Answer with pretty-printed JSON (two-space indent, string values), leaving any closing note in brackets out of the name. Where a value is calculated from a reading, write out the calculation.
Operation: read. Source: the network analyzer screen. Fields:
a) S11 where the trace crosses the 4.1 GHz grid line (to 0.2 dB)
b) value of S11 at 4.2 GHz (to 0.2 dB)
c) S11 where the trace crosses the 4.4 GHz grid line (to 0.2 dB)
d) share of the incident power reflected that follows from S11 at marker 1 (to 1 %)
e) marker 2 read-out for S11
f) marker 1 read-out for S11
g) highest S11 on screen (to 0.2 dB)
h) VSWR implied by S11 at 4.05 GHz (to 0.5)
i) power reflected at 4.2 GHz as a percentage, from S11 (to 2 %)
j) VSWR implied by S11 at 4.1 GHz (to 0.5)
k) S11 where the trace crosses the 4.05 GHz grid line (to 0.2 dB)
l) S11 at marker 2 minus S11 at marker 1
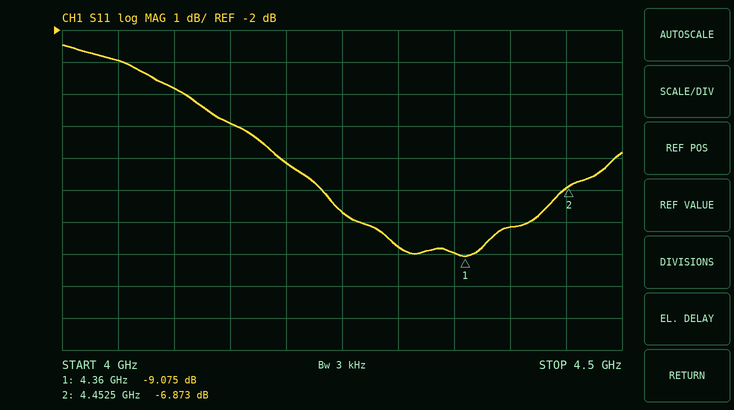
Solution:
{
  "S11 where the trace crosses the 4.1 GHz grid line": "-3.8 dB",
  "value of S11 at 4.2 GHz": "-6.2 dB",
  "S11 where the trace crosses the 4.4 GHz grid line": "-8.2 dB",
  "share of the incident power reflected that follows from S11 at marker 1": "10^(-9.075/10) ≈ 12 %",
  "marker 2 read-out for S11": "-6.873 dB",
  "marker 1 read-out for S11": "-9.075 dB",
  "highest S11 on screen": "-2.4 dB",
  "VSWR implied by S11 at 4.05 GHz": "|Γ| = 10^(-3/20) = 0.7079; VSWR = (1 + 0.7079)/(1 − 0.7079) ≈ 5.85, so 6.0 to the nearest 0.5",
  "power reflected at 4.2 GHz as a percentage, from S11": "10^(-6.2/10) ≈ 24 %",
  "VSWR implied by S11 at 4.1 GHz": "|Γ| = 10^(-3.8/20) = 0.6457; VSWR = (1 + 0.6457)/(1 − 0.6457) ≈ 4.64, so 4.5 to the nearest 0.5",
  "S11 where the trace crosses the 4.05 GHz grid line": "-3.0 dB",
  "S11 at marker 2 minus S11 at marker 1": "-6.873 − (-9.075) = 2.202 dB"
}
